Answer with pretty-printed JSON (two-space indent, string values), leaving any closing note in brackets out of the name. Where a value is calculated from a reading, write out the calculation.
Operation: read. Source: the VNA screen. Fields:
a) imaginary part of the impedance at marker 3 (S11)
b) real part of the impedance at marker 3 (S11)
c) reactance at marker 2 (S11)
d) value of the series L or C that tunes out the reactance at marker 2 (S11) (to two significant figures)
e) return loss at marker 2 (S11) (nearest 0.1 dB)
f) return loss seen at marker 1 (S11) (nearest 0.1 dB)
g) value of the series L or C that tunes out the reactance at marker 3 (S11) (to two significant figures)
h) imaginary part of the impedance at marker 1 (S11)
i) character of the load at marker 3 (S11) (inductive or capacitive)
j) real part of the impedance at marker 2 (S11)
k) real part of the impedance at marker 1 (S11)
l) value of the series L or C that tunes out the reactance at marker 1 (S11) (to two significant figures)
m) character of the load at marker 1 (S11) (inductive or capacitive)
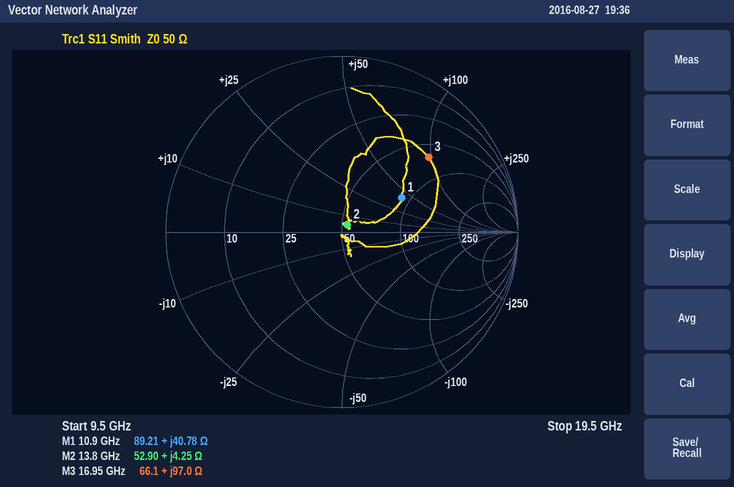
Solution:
{
  "imaginary part of the impedance at marker 3": "+97.0 Ω",
  "real part of the impedance at marker 3": "66.1 Ω",
  "reactance at marker 2": "+4.25 Ω",
  "value of the series L or C that tunes out the reactance at marker 2 (S11)": "C = 1/(2π × 13.8 GHz × 4.25 Ω) ≈ 2.7 pF",
  "return loss at marker 2 (S11)": "26.0 dB",
  "return loss seen at marker 1 (S11)": "8.2 dB",
  "value of the series L or C that tunes out the reactance at marker 3 (S11)": "C = 1/(2π × 16.95 GHz × 97 Ω) ≈ 97 fF",
  "imaginary part of the impedance at marker 1": "+40.78 Ω",
  "character of the load at marker 3 (S11)": "inductive",
  "real part of the impedance at marker 2": "52.90 Ω",
  "real part of the impedance at marker 1": "89.21 Ω",
  "value of the series L or C that tunes out the reactance at marker 1 (S11)": "C = 1/(2π × 10.9 GHz × 40.78 Ω) ≈ 358 fF, so 360 fF to two significant figures",
  "character of the load at marker 1 (S11)": "inductive"
}
